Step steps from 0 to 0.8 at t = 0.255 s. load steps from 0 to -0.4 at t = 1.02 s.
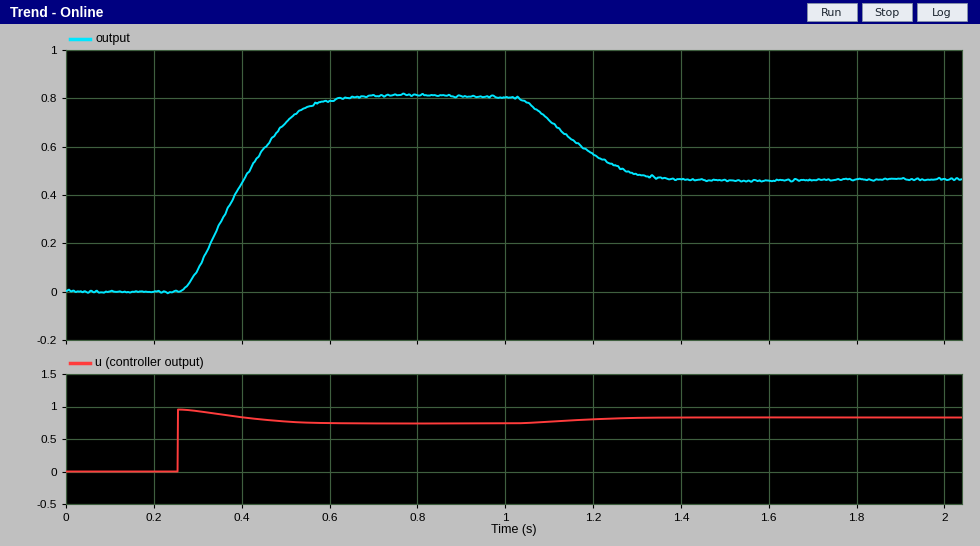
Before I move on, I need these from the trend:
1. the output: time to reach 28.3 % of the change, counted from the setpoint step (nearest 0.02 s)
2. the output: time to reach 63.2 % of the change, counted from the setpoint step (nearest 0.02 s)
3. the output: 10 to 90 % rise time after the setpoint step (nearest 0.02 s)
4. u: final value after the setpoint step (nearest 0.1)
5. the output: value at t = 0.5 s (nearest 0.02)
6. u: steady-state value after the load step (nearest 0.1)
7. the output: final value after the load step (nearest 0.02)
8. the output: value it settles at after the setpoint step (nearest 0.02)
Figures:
0.08 s
0.16 s
0.22 s
0.7
0.70
0.8
0.46
0.80
